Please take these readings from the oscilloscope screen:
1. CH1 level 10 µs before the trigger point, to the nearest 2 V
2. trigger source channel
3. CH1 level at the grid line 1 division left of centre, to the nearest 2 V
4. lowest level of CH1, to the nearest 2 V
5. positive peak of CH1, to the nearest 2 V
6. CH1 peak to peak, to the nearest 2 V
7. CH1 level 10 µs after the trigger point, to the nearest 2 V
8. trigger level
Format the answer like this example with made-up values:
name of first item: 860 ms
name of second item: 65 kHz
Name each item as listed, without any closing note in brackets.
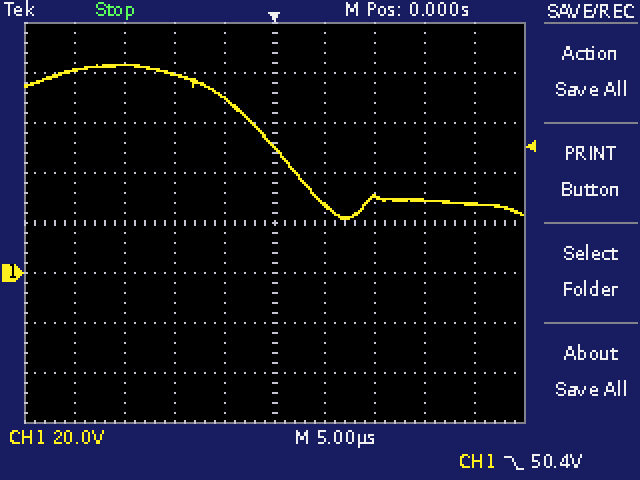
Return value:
CH1 level 10 µs before the trigger point, to the nearest 2 V: 80 V
trigger source channel: CH1
CH1 level at the grid line 1 division left of centre, to the nearest 2 V: 70 V
lowest level of CH1, to the nearest 2 V: 22 V
positive peak of CH1, to the nearest 2 V: 84 V
CH1 peak to peak, to the nearest 2 V: 62 V
CH1 level 10 µs after the trigger point, to the nearest 2 V: 30 V
trigger level: 50.4 V
